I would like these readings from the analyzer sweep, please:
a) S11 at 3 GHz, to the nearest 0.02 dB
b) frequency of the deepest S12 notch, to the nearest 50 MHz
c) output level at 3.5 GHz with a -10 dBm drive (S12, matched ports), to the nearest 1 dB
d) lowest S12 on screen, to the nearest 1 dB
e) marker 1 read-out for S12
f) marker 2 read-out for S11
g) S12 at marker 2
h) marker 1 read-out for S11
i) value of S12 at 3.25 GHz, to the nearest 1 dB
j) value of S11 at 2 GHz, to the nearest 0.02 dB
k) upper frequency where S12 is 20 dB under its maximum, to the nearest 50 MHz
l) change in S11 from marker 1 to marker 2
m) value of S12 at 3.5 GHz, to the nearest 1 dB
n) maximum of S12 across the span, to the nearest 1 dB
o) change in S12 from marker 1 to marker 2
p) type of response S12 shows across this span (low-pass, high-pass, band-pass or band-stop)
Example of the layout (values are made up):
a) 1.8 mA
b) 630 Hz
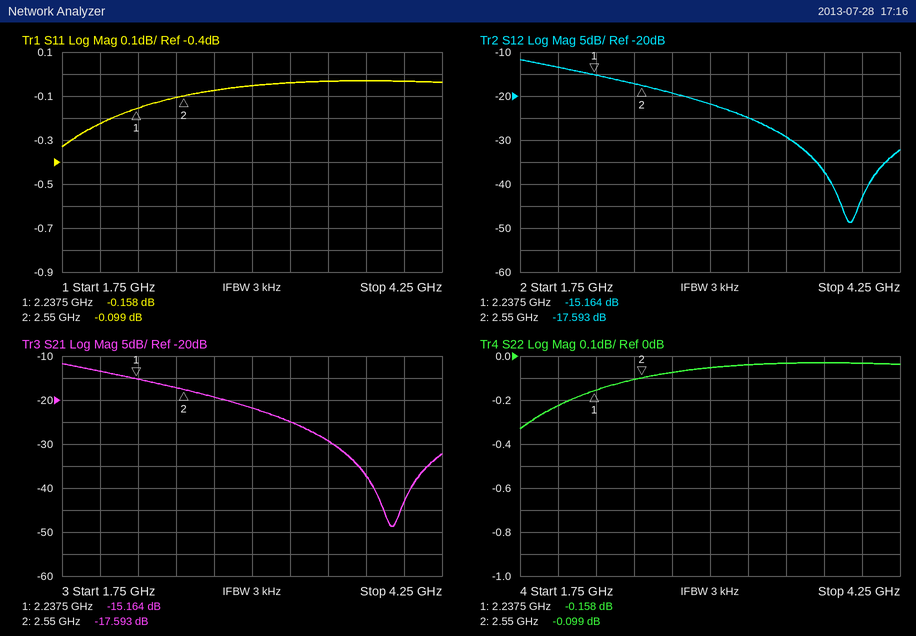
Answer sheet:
a) -0.06 dB
b) 3.90 GHz
c) -39 dBm
d) -49 dB
e) -15.164 dB
f) -0.099 dB
g) -17.593 dB
h) -0.158 dB
i) -25 dB
j) -0.22 dB
k) 3.60 GHz
l) 0.059 dB
m) -29 dB
n) -12 dB
o) -2.429 dB
p) low-pass
